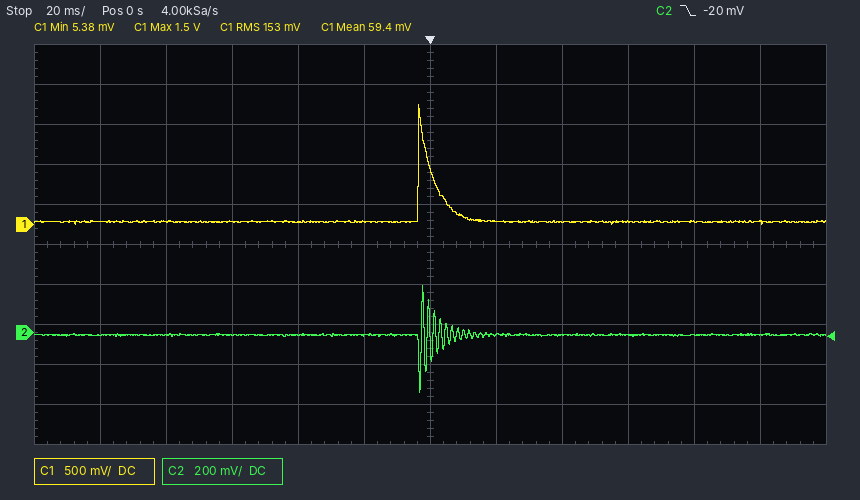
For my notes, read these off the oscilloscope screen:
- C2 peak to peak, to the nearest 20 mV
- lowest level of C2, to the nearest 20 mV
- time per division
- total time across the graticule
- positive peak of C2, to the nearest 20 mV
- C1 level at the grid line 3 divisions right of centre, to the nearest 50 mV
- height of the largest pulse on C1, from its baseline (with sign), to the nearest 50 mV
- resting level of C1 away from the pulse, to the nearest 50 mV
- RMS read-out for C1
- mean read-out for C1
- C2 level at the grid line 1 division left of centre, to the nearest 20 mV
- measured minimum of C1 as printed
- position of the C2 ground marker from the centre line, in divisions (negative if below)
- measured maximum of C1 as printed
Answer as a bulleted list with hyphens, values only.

- 540 mV
- -300 mV
- 20 ms
- 240 ms
- 240 mV
- 50 mV
- +1.45 V
- 50 mV
- 153 mV
- 59.4 mV
- -20 mV
- 5.38 mV
- -2.2 div
- 1.5 V
